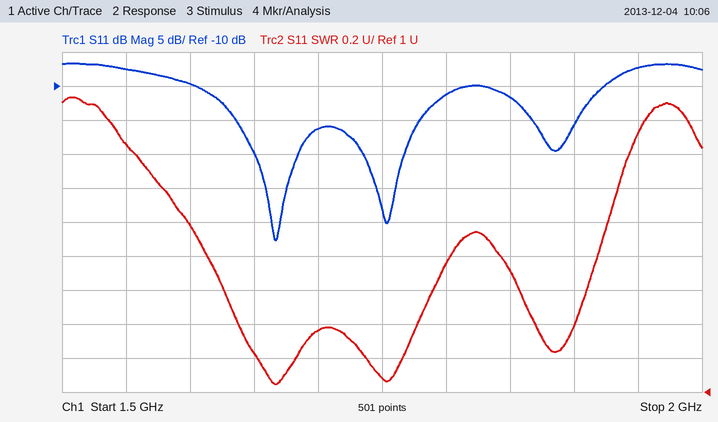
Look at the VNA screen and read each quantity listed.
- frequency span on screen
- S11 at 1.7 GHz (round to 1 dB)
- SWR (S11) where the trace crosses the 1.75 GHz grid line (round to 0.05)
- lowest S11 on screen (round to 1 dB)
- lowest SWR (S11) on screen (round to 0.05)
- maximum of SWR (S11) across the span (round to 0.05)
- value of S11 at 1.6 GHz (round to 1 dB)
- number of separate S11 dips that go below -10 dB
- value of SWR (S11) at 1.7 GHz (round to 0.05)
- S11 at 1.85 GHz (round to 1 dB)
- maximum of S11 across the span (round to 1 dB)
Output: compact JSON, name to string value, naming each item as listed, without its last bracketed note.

{"frequency span on screen": "500 MHz", "S11 at 1.7 GHz": "-16 dB", "SWR (S11) where the trace crosses the 1.75 GHz grid line": "1.10", "lowest S11 on screen": "-33 dB", "lowest SWR (S11) on screen": "1.05", "maximum of SWR (S11) across the span": "2.75", "value of S11 at 1.6 GHz": "-10 dB", "number of separate S11 dips that go below -10 dB": "3", "value of SWR (S11) at 1.7 GHz": "1.35", "S11 at 1.85 GHz": "-12 dB", "maximum of S11 across the span": "-7 dB"}
